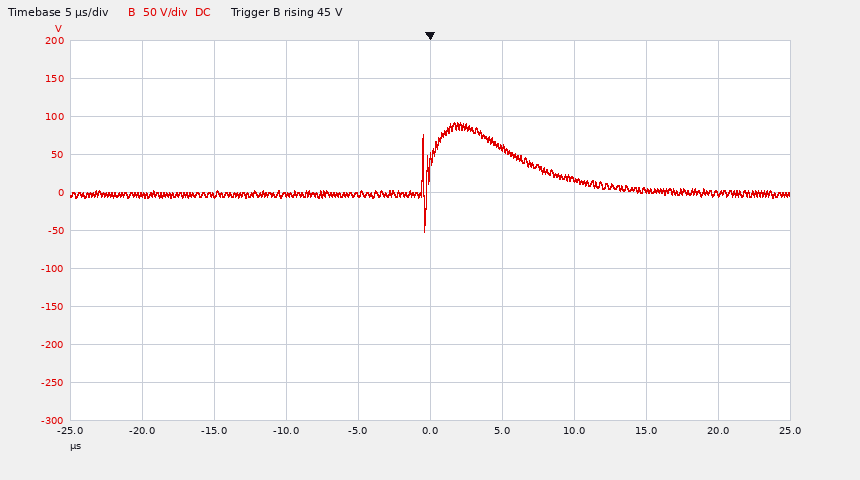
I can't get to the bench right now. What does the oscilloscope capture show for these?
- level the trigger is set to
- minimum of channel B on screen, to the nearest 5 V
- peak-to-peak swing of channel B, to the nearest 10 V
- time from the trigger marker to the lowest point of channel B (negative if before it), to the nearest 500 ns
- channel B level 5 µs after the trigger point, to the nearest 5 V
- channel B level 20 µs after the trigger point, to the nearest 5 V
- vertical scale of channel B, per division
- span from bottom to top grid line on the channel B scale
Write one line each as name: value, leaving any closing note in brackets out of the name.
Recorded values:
level the trigger is set to: 45 V
minimum of channel B on screen, to the nearest 5 V: -50 V
peak-to-peak swing of channel B, to the nearest 10 V: 140 V
time from the trigger marker to the lowest point of channel B (negative if before it), to the nearest 500 ns: -500 ns
channel B level 5 µs after the trigger point, to the nearest 5 V: 60 V
channel B level 20 µs after the trigger point, to the nearest 5 V: 0 V
vertical scale of channel B, per division: 50 V
span from bottom to top grid line on the channel B scale: 500 V
